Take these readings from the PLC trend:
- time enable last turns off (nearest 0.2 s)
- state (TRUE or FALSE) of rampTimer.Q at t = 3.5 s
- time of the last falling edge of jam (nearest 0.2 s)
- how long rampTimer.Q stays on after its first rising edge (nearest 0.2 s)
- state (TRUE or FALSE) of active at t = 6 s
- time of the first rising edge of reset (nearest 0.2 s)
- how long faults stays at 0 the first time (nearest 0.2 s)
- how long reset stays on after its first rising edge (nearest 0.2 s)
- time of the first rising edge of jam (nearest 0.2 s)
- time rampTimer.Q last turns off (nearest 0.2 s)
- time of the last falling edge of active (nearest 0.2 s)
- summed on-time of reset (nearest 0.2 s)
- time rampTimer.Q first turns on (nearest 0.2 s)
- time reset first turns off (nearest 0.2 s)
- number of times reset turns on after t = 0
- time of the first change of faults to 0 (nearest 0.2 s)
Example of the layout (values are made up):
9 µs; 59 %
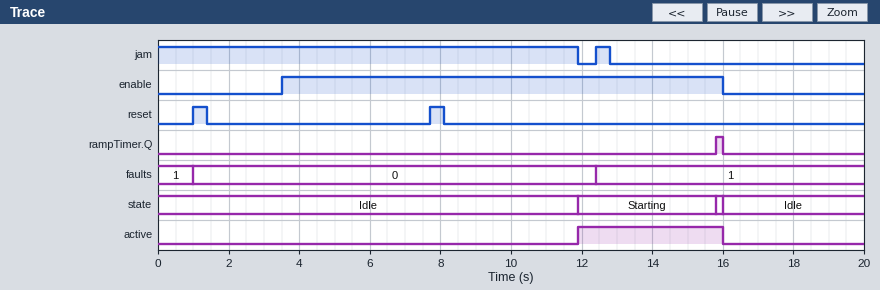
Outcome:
16.0 s; FALSE; 12.8 s; 0.2 s; FALSE; 1.0 s; 11.4 s; 0.4 s; 12.4 s; 16.0 s; 16.0 s; 0.8 s; 15.8 s; 1.4 s; 2; 1.0 s
